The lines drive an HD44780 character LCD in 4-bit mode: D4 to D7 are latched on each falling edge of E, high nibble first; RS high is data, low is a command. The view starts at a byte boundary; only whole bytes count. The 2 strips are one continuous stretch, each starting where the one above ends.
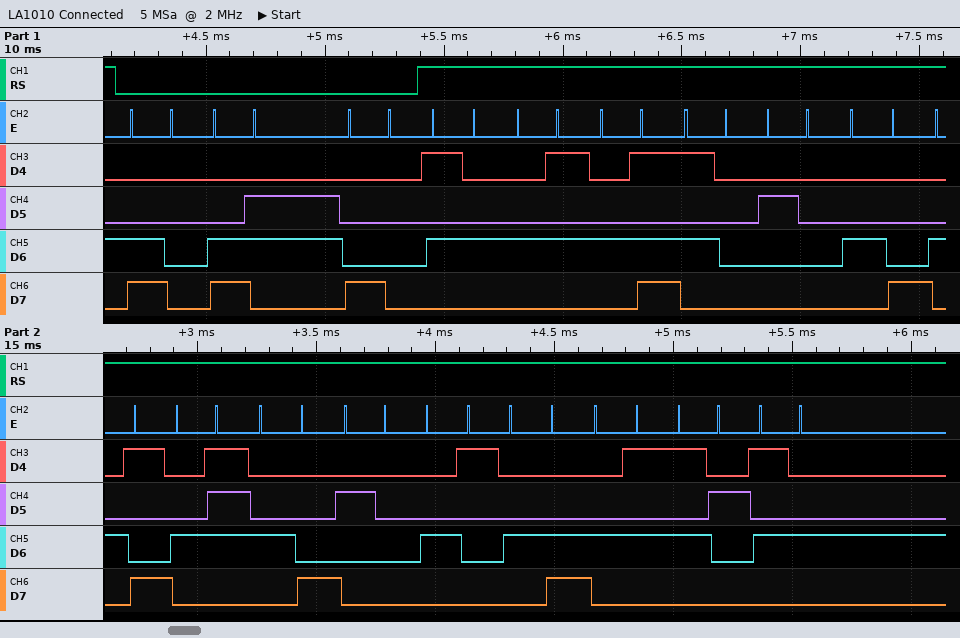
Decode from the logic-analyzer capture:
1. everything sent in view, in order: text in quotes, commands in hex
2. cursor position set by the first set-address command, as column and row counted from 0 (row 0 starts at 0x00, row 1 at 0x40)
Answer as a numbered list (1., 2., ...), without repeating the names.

1. 0xC0 0xC6 0x80 "TEMP HIGH ALERT"
2. column 0, row 1
